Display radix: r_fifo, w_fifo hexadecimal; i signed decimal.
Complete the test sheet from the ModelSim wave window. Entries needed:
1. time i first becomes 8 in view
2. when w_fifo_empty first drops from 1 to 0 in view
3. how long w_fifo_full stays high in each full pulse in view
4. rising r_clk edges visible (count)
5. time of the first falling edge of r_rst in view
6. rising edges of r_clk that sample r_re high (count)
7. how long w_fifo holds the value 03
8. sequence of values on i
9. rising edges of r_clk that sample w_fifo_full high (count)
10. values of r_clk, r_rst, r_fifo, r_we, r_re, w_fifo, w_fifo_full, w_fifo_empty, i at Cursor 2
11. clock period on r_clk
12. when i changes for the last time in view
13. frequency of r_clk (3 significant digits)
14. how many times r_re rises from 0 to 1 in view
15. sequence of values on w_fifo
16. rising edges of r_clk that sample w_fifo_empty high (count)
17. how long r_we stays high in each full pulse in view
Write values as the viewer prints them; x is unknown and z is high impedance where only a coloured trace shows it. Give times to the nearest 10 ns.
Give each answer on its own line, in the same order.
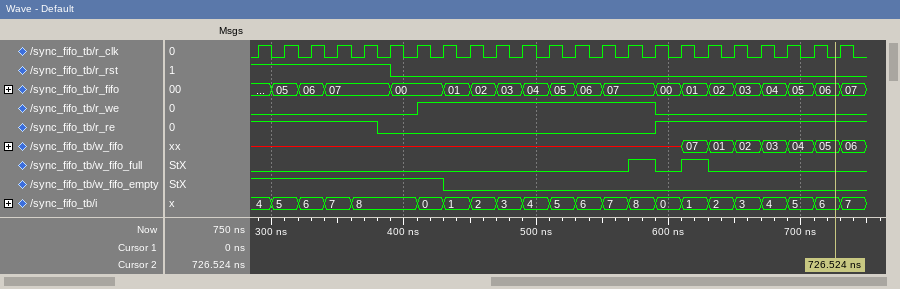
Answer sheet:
360 ns
430 ns
20 ns, 20 ns
23
390 ns
12
20 ns
4, 5, 6, 7, 8, 0, 1, 2, 3, 4, 5, 6, 7, 8, 0, 1, 2, 3, 4, 5, 6, 7
2
r_clk=0, r_rst=0, r_fifo=06, r_we=0, r_re=1, w_fifo=05, w_fifo_full=0, w_fifo_empty=0, i=6
20 ns
730 ns
50.0 MHz
1
x, 07, 01, 02, 03, 04, 05, 06
8
180 ns
